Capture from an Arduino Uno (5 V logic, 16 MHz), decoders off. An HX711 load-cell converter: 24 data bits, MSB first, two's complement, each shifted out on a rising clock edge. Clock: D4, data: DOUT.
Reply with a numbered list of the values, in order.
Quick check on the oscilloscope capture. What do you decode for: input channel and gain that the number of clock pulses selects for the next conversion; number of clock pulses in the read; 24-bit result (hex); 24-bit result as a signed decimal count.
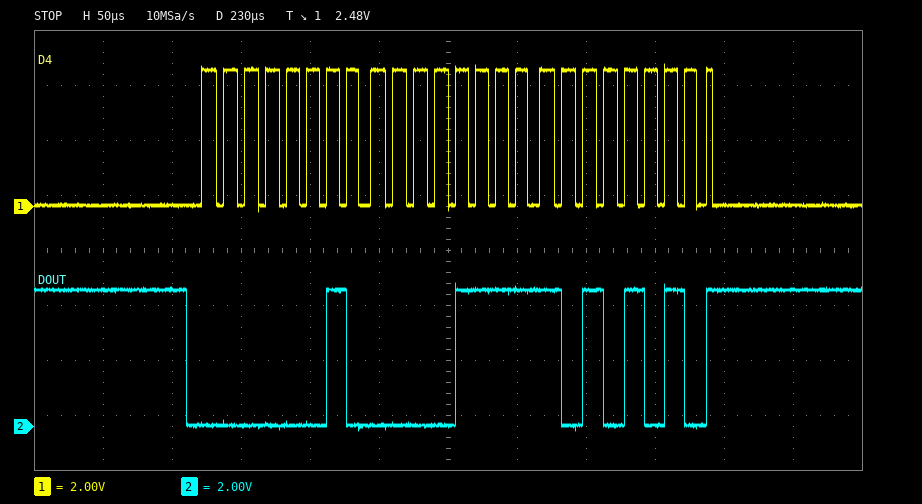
1. channel A, gain 128
2. 25
3. 0x020FAA
4. 135082
